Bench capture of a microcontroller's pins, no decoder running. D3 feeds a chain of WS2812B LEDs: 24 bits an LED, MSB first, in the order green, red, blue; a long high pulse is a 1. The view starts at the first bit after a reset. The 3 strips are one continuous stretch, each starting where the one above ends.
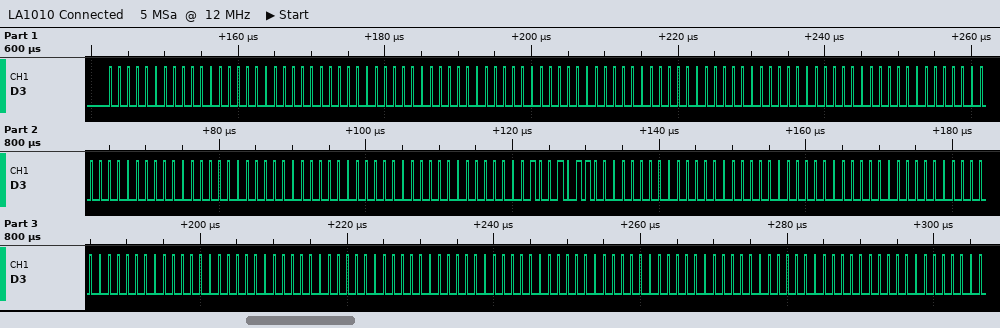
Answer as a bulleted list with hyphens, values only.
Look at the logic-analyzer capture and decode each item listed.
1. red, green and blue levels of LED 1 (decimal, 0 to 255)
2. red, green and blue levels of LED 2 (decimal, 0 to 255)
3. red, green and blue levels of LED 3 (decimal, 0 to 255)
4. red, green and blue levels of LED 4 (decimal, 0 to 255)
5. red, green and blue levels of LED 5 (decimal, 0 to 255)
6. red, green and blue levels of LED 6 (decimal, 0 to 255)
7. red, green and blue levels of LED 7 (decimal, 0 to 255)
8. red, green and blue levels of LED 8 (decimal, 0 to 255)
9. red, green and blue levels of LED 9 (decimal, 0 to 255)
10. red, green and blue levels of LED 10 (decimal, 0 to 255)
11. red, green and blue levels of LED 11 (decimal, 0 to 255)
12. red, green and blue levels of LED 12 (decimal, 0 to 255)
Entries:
- 0, 0, 0
- 0, 0, 0
- 0, 0, 0
- 0, 0, 0
- 0, 0, 0
- 0, 0, 0
- 0, 150, 0
- 0, 0, 0
- 0, 0, 0
- 0, 0, 0
- 0, 0, 0
- 0, 0, 0
